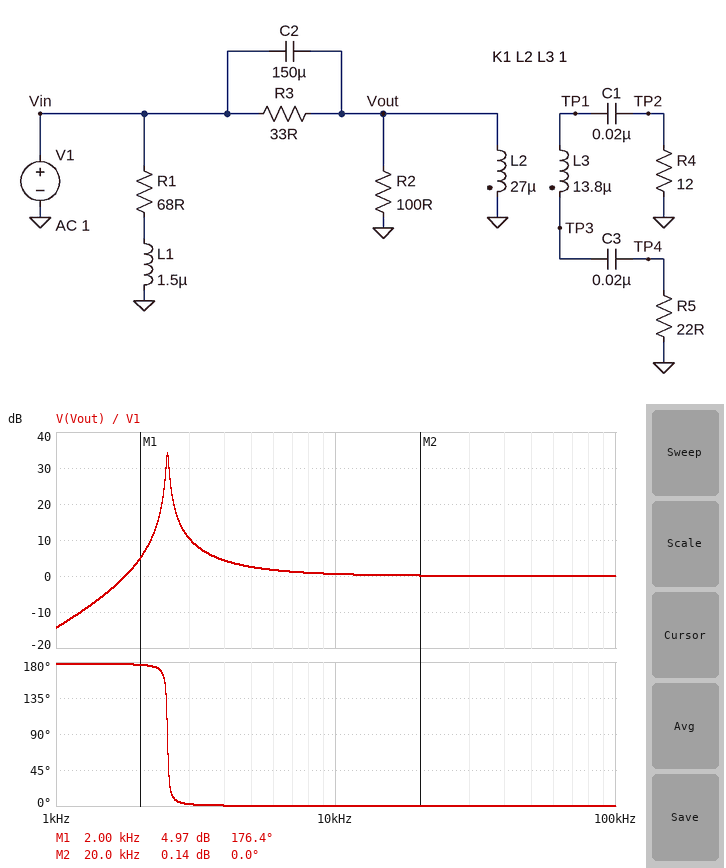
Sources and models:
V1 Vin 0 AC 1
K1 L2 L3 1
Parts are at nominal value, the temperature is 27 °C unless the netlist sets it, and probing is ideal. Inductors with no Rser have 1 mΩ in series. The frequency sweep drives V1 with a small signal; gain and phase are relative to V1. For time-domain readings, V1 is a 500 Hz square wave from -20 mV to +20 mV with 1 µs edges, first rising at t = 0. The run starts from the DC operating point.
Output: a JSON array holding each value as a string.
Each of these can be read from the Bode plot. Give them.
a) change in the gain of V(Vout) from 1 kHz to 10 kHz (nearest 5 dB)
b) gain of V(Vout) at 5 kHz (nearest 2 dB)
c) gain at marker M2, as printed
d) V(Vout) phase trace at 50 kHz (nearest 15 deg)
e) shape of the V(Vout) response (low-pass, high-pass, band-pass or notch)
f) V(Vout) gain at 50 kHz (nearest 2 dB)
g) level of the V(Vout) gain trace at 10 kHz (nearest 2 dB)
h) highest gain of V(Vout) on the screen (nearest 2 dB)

["15 dB", "2 dB", "0.14 dB", "0 deg", "high-pass", "0 dB", "0 dB", "34 dB"]
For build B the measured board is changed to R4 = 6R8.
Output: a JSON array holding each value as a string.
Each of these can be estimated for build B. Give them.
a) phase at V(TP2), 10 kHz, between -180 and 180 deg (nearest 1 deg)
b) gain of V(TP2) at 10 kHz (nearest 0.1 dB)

["89 deg", "-49.7 dB"]
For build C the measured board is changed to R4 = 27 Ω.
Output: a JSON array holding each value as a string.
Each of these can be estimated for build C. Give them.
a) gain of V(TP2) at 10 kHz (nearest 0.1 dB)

["-37.8 dB"]
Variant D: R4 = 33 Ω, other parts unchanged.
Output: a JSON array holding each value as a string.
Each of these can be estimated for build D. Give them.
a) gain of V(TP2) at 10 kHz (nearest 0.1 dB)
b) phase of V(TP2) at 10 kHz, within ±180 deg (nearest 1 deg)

["-36.0 dB", "88 deg"]
